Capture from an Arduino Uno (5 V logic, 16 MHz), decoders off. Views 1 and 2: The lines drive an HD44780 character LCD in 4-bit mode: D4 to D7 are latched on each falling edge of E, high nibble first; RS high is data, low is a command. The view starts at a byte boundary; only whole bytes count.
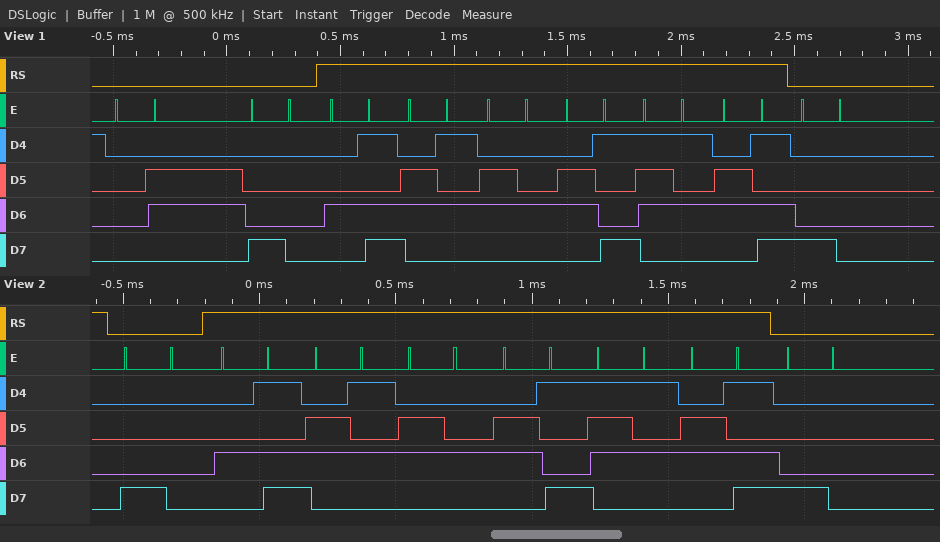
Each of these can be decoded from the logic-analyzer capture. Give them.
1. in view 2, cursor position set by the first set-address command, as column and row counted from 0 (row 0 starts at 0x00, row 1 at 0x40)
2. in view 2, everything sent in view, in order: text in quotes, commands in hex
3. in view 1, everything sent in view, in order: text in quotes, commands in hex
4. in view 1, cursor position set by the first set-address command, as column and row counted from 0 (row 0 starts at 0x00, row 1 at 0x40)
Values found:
column 0, row 0
0x80 "Medium" 0x80
0x06 0x80 "Medium" 0x80
column 0, row 0
